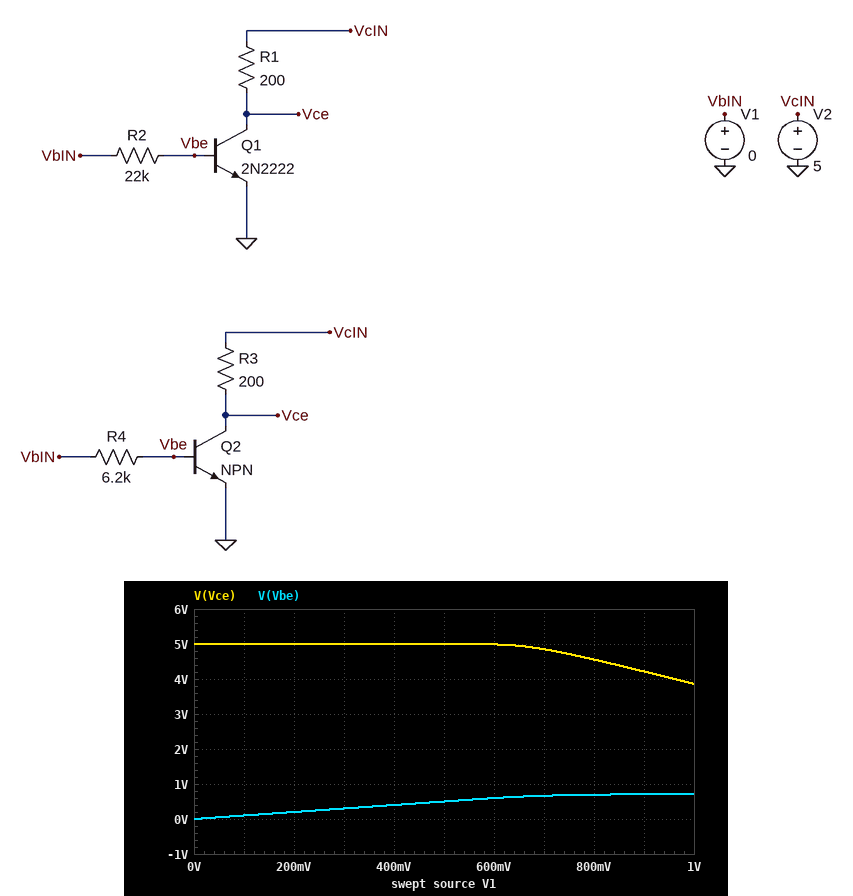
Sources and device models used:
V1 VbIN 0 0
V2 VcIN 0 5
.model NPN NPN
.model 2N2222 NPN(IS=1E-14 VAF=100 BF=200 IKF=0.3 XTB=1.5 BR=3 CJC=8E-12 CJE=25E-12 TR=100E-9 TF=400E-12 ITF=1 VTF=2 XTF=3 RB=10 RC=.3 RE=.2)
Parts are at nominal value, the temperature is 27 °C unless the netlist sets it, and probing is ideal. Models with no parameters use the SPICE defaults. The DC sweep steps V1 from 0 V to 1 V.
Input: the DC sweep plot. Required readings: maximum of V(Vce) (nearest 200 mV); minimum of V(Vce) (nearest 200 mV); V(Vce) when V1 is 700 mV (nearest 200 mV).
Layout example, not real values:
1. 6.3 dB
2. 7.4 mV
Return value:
1. 5.0 V
2. 3.8 V
3. 4.8 V
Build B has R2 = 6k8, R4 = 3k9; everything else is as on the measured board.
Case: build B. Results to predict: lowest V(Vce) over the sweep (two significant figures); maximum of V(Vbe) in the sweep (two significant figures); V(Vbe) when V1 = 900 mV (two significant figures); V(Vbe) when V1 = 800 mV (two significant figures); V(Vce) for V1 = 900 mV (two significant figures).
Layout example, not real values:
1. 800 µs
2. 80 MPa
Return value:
1. 3.0 V
2. 740 mV
3. 730 mV
4. 710 mV
5. 3.6 V
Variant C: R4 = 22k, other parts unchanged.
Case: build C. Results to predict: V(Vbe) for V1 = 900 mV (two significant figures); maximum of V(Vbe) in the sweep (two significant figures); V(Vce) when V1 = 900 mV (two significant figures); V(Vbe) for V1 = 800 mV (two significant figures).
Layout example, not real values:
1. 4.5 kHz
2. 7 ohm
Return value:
1. 690 mV
2. 700 mV
3. 4.6 V
4. 680 mV
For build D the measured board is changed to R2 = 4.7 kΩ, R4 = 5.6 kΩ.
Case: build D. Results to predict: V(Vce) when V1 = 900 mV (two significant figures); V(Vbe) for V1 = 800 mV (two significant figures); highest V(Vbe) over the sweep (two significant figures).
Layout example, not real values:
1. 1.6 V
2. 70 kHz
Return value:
1. 3.7 V
2. 710 mV
3. 740 mV
